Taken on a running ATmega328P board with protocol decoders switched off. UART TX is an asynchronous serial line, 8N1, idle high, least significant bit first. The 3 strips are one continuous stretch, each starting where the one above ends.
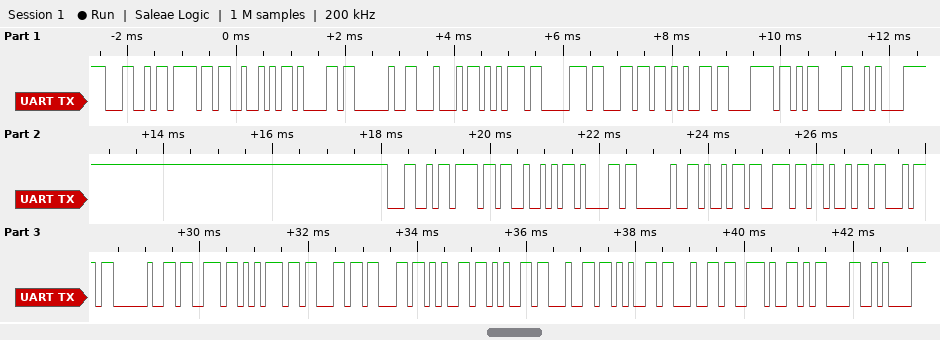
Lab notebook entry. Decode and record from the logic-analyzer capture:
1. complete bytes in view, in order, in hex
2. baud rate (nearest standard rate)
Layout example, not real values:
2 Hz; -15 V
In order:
4C 6F 52 61 20 44 75 70 6C 65 78 0D 0A 4C 6F 52 61 20 69 6E 69 74 20 73 75 63 63 65 65 64 65 64 2E 0D 0A; 9600 baud
